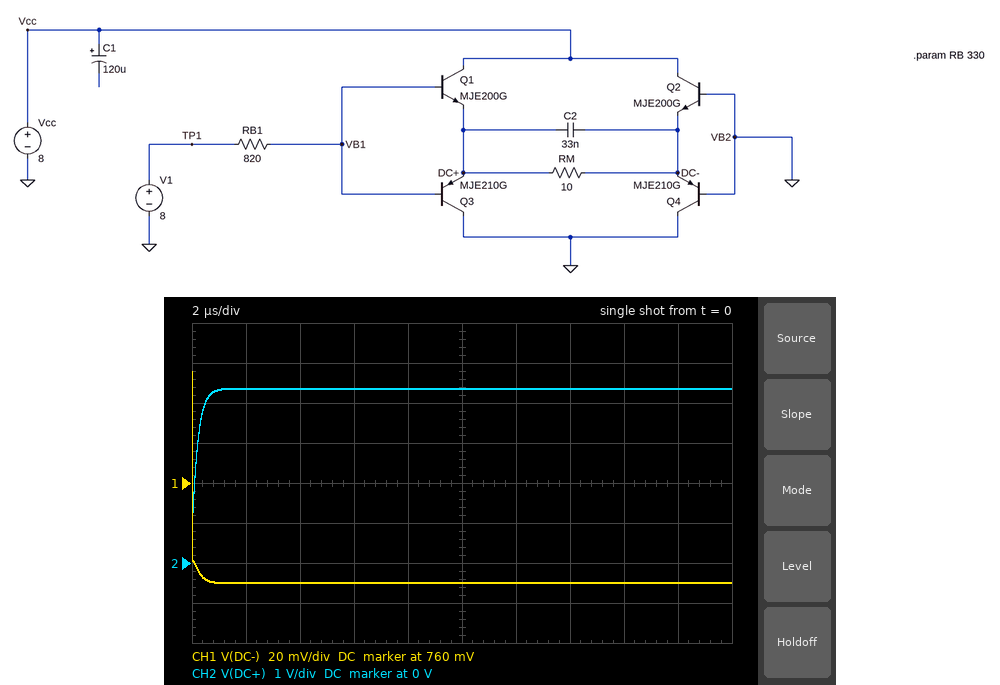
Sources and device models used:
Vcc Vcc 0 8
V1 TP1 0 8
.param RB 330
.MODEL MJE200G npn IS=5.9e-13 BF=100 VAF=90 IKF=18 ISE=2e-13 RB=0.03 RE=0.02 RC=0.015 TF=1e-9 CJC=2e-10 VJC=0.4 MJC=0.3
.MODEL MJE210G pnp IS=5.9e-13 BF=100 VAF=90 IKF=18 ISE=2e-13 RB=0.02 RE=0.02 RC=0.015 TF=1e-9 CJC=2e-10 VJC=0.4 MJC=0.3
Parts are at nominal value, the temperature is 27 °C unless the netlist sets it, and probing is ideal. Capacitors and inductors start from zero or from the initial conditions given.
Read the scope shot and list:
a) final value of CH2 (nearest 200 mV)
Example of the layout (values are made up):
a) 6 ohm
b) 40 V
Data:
a) 4.4 V
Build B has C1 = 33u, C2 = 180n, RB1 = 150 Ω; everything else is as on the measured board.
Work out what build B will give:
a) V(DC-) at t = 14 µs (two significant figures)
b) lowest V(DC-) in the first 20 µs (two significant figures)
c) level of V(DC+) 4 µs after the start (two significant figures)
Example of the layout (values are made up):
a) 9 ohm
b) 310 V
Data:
a) 730 mV
b) 720 mV
c) 6.4 V
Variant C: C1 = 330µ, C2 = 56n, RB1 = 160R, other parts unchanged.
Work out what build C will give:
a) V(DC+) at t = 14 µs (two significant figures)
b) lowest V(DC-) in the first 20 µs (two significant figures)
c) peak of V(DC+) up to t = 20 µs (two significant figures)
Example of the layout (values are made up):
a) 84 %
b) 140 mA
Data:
a) 6.4 V
b) 720 mV
c) 6.6 V
